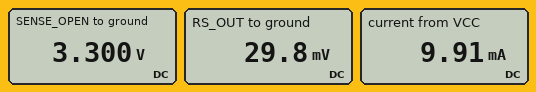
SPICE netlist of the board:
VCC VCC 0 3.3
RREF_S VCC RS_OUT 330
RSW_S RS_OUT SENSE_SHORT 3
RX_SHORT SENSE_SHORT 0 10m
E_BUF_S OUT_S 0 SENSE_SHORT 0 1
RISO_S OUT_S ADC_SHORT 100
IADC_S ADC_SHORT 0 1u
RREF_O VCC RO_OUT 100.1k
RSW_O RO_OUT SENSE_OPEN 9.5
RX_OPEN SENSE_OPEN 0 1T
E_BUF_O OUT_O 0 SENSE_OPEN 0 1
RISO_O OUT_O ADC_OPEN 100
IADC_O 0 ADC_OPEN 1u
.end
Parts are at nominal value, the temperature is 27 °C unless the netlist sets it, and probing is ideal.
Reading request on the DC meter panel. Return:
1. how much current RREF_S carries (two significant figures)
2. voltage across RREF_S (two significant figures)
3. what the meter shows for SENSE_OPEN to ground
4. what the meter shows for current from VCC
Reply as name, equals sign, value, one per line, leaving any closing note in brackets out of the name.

how much current RREF_S carries = 9.9 mA
voltage across RREF_S = 3.3 V
what the meter shows for SENSE_OPEN to ground = 3.300 V
what the meter shows for current from VCC = 9.91 mA
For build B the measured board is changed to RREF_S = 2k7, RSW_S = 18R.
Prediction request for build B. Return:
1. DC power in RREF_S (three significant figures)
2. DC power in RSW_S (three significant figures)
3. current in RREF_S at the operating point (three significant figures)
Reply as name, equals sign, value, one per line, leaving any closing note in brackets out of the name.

DC power in RREF_S = 3.98 mW
DC power in RSW_S = 26.5 µW
current in RREF_S at the operating point = 1.21 mA
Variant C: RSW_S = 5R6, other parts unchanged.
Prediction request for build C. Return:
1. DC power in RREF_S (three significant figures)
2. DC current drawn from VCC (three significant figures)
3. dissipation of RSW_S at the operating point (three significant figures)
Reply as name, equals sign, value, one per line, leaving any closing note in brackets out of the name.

DC power in RREF_S = 31.9 mW
DC current drawn from VCC = 9.83 mA
dissipation of RSW_S at the operating point = 541 µW
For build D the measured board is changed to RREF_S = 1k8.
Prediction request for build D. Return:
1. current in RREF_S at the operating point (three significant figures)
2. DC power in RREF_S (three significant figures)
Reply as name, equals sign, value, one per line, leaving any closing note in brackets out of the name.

current in RREF_S at the operating point = 1.83 mA
DC power in RREF_S = 6.03 mW
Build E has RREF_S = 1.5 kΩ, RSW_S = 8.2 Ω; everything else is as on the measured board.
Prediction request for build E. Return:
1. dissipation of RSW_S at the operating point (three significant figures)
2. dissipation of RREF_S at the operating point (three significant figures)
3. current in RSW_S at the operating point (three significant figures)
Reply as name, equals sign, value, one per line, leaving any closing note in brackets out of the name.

dissipation of RSW_S at the operating point = 39.3 µW
dissipation of RREF_S at the operating point = 7.18 mW
current in RSW_S at the operating point = 2.19 mA
